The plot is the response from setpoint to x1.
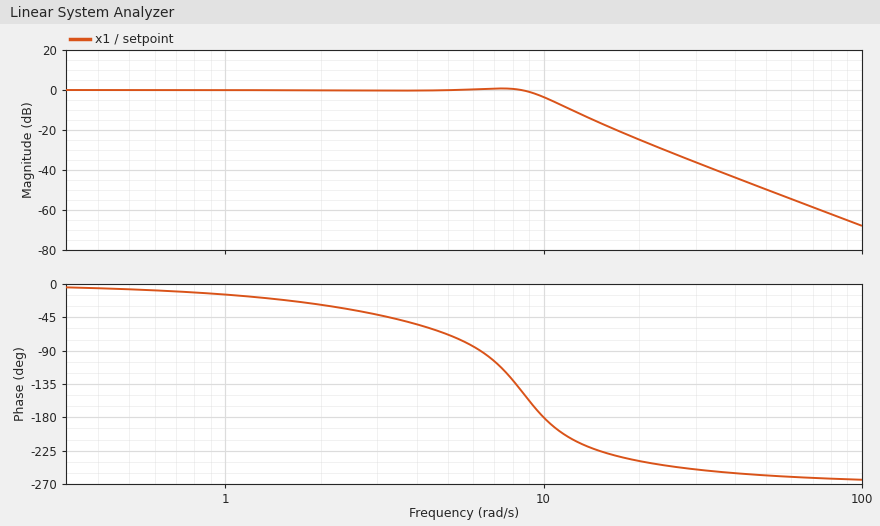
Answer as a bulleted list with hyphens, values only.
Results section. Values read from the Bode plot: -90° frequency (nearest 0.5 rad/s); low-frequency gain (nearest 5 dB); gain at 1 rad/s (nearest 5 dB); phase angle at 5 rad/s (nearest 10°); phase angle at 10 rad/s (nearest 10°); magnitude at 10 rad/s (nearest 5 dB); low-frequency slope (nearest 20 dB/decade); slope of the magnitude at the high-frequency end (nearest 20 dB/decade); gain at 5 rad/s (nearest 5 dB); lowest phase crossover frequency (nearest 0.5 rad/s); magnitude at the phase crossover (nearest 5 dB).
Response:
- 6.5 rad/s
- 0 dB
- 0 dB
- -70°
- -180°
- -5 dB
- 0 dB/decade
- -60 dB/decade
- 0 dB
- 10.0 rad/s
- -5 dB
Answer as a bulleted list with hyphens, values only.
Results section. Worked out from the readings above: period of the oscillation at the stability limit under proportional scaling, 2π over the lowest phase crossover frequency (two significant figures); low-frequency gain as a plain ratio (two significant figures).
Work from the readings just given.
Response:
- 0.63 s
- 1.0
